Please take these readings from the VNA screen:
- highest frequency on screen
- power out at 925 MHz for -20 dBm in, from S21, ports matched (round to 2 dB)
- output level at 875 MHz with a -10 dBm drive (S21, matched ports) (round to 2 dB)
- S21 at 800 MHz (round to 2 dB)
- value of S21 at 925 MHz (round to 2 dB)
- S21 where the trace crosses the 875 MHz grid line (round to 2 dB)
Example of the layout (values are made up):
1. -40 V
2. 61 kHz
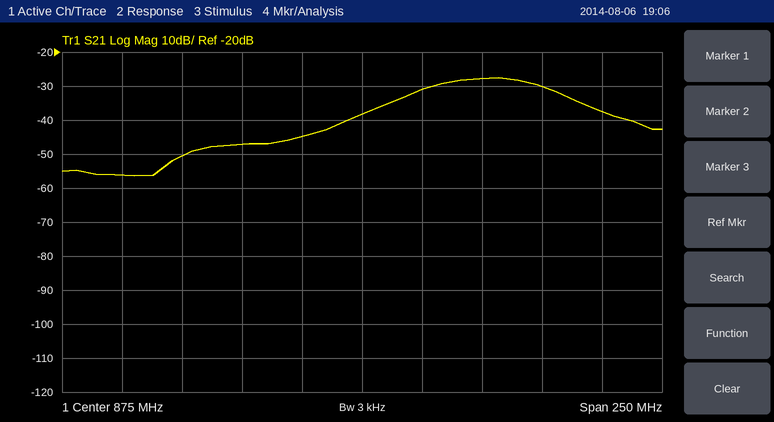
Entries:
1. 1 GHz
2. -48 dBm
3. -48 dBm
4. -50 dB
5. -28 dB
6. -38 dB
